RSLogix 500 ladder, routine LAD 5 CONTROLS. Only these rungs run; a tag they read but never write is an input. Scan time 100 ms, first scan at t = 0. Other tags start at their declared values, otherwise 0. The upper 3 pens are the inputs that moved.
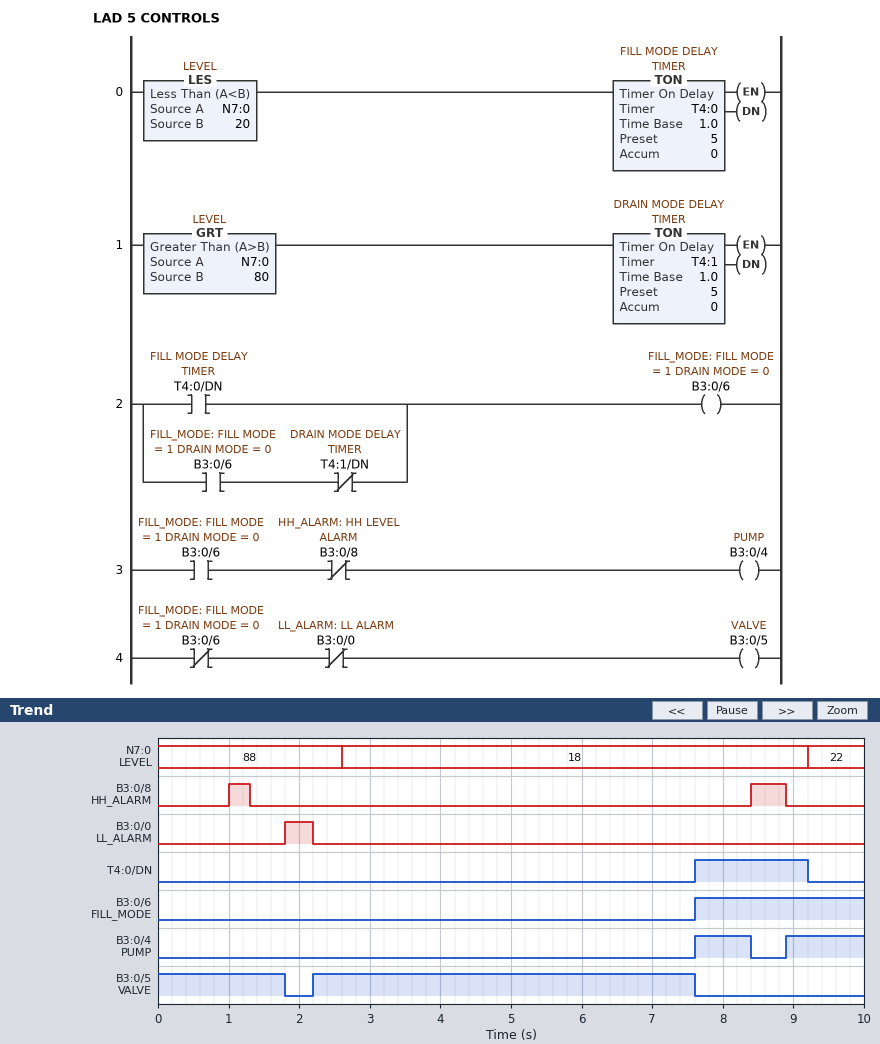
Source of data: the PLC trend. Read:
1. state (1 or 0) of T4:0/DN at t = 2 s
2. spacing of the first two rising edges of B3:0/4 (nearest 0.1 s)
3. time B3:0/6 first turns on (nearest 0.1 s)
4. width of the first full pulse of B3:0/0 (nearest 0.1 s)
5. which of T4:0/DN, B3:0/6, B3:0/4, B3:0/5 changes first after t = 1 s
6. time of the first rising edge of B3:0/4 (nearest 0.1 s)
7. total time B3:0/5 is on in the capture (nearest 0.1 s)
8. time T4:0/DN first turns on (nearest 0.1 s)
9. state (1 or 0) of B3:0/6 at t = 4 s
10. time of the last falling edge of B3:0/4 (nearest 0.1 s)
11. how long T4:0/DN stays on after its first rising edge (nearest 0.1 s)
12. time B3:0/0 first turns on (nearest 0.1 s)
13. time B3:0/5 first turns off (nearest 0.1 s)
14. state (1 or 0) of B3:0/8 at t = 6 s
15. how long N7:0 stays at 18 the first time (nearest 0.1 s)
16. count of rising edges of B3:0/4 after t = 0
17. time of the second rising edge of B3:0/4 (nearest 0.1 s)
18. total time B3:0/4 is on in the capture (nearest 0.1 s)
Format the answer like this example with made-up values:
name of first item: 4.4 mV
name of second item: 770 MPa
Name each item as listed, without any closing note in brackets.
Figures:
state (1 or 0) of T4:0/DN at t = 2 s: 0
spacing of the first two rising edges of B3:0/4: 1.3 s
time B3:0/6 first turns on: 7.6 s
width of the first full pulse of B3:0/0: 0.4 s
which of T4:0/DN, B3:0/6, B3:0/4, B3:0/5 changes first after t = 1 s: B3:0/5
time of the first rising edge of B3:0/4: 7.6 s
total time B3:0/5 is on in the capture: 7.2 s
time T4:0/DN first turns on: 7.6 s
state (1 or 0) of B3:0/6 at t = 4 s: 0
time of the last falling edge of B3:0/4: 8.4 s
how long T4:0/DN stays on after its first rising edge: 1.6 s
time B3:0/0 first turns on: 1.8 s
time B3:0/5 first turns off: 1.8 s
state (1 or 0) of B3:0/8 at t = 6 s: 0
how long N7:0 stays at 18 the first time: 6.6 s
count of rising edges of B3:0/4 after t = 0: 2
time of the second rising edge of B3:0/4: 8.9 s
total time B3:0/4 is on in the capture: 1.9 s
